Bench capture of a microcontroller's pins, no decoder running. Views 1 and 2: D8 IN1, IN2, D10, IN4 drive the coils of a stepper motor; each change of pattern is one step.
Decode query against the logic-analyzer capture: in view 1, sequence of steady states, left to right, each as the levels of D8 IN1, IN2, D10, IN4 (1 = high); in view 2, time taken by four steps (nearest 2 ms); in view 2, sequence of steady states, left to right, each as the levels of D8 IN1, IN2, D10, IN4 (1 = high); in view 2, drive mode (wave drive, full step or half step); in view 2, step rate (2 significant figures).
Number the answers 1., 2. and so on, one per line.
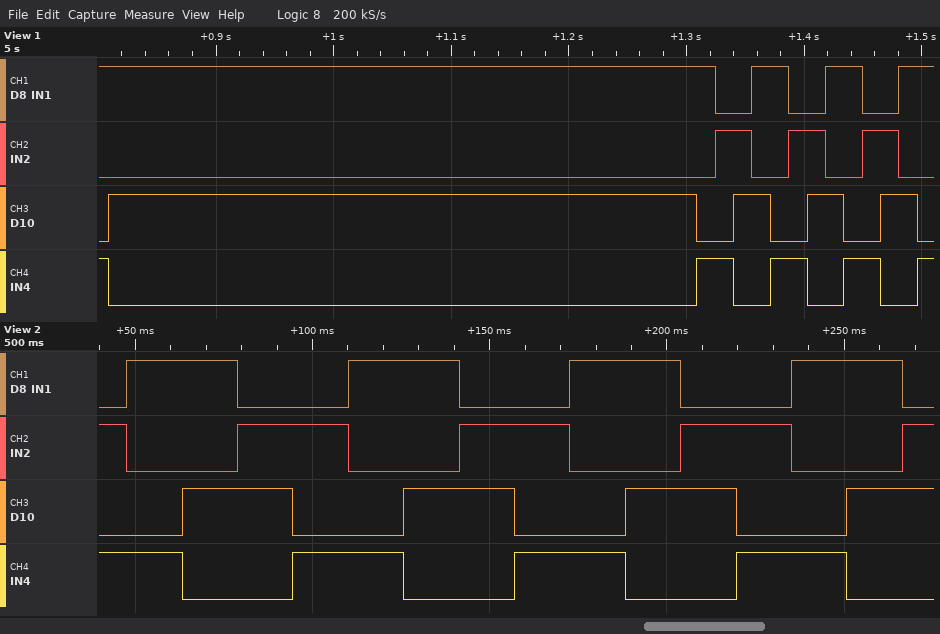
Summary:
1. 1001 1010 1001 0101 0110 1010 1001 0101 0110 1010 1001 0101 0110 1010 1001
2. 62 ms
3. 0101 1001 1010 0110 0101 1001 1010 0110 0101 1001 1010 0110 0101 1001 1010 0110
4. full step
5. 64 steps/s
